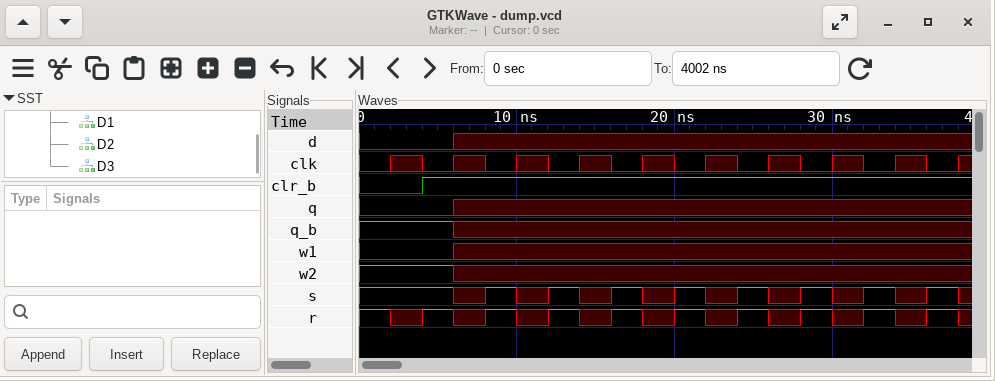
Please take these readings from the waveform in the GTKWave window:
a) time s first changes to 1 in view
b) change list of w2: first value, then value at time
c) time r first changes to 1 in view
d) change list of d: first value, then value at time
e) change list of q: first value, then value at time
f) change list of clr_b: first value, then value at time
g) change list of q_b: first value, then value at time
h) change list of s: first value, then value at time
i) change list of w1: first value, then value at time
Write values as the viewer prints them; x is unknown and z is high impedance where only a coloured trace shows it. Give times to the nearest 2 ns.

8 ns
1, x at 6 ns
4 ns
0, x at 6 ns
0, x at 6 ns
0, 1 at 4 ns
1, x at 6 ns
1, x at 6 ns, 1 at 8 ns, x at 10 ns, 1 at 12 ns, x at 14 ns, 1 at 16 ns, x at 18 ns, 1 at 20 ns, x at 22 ns, 1 at 24 ns, x at 26 ns, 1 at 28 ns, x at 30 ns, 1 at 32 ns, x at 34 ns, 1 at 36 ns, x at 38 ns
0, x at 6 ns
